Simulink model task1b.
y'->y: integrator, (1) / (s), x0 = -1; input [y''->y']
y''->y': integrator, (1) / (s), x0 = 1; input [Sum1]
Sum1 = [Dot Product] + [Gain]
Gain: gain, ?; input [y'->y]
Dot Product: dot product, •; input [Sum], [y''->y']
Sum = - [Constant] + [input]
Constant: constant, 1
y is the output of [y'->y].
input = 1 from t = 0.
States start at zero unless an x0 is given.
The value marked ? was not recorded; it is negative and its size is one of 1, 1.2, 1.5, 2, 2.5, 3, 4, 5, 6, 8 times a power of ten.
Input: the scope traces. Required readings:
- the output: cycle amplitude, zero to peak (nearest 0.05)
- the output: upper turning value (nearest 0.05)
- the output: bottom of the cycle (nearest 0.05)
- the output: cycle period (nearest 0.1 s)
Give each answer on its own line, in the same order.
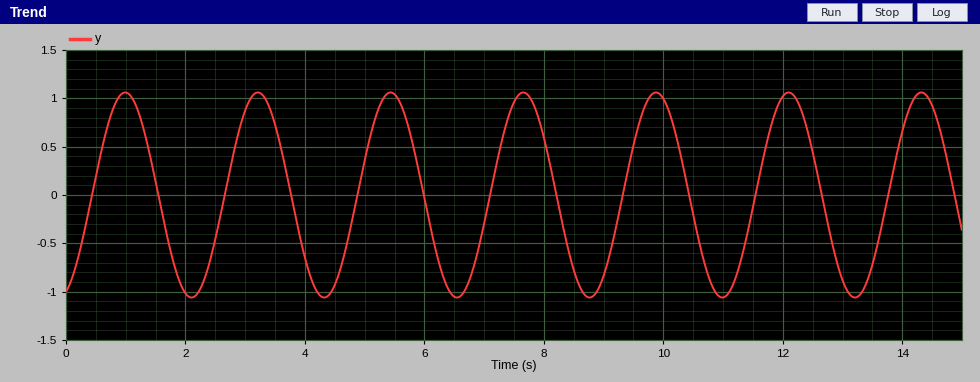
1.05
1.05
-1.05
2.2 s
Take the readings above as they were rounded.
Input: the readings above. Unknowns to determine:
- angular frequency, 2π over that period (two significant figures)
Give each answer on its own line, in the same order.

2.9 rad/s
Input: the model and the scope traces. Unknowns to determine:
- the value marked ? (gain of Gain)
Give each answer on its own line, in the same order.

-8
